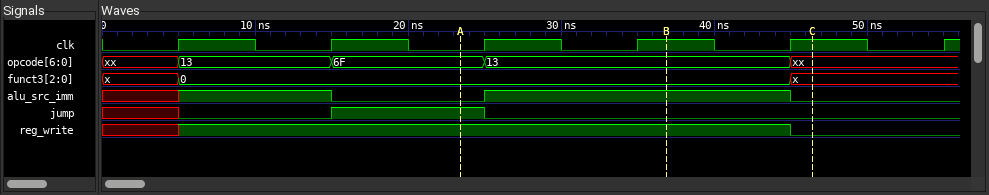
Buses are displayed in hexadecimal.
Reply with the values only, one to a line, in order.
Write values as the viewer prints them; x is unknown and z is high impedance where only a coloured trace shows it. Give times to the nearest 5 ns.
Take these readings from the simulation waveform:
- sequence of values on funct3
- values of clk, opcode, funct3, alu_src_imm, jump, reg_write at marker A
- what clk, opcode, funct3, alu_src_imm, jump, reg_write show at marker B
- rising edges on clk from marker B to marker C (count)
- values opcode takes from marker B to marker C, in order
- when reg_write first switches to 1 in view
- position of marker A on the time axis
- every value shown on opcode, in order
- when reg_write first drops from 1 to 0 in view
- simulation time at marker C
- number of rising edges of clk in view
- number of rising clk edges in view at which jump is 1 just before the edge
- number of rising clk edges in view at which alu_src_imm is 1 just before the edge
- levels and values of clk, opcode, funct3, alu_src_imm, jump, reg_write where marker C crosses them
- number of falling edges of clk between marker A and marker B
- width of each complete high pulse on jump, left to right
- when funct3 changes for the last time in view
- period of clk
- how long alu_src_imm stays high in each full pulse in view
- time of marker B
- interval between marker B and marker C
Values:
x, 0, x
clk=0, opcode=6F, funct3=0, alu_src_imm=0, jump=1, reg_write=1
clk=1, opcode=13, funct3=0, alu_src_imm=1, jump=0, reg_write=1
1
13, xx
5 ns
25 ns
xx, 13, 6F, 13, xx
45 ns
45 ns
6
1
3
clk=1, opcode=xx, funct3=x, alu_src_imm=0, jump=0, reg_write=0
1
10 ns
45 ns
10 ns
20 ns
35 ns
10 ns
